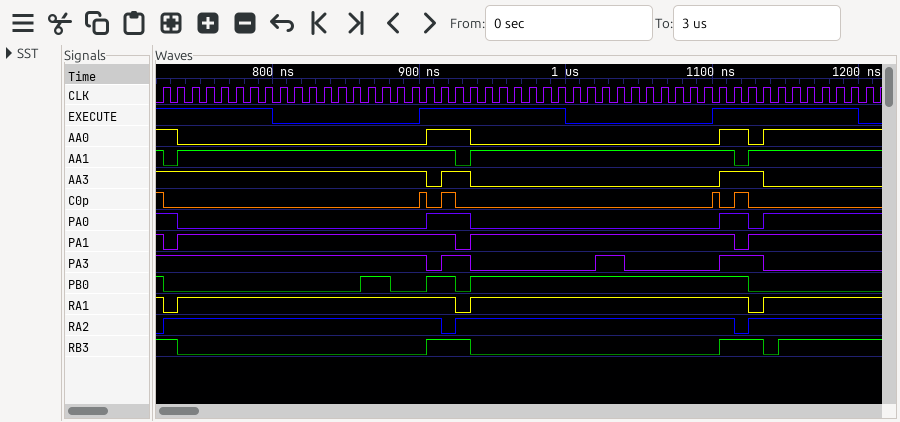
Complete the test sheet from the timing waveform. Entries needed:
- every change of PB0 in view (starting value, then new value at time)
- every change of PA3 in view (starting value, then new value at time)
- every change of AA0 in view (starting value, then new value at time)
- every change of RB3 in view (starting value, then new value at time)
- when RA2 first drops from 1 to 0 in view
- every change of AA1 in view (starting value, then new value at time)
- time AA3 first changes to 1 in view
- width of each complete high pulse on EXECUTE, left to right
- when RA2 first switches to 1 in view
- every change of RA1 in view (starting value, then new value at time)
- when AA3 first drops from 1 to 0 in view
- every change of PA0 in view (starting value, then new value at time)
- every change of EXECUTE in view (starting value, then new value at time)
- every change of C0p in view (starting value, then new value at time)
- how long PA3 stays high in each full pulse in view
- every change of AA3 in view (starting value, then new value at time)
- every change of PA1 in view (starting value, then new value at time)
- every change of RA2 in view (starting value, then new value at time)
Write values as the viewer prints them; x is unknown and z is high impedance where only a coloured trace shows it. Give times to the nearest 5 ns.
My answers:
1, 0 at 725 ns, 1 at 860 ns, 0 at 880 ns, 1 at 905 ns, 0 at 925 ns, 1 at 935 ns, 0 at 1125 ns
1, 0 at 905 ns, 1 at 915 ns, 0 at 935 ns, 1 at 1020 ns, 0 at 1040 ns, 1 at 1105 ns, 0 at 1135 ns
1, 0 at 735 ns, 1 at 905 ns, 0 at 935 ns, 1 at 1105 ns, 0 at 1125 ns, 1 at 1135 ns
1, 0 at 735 ns, 1 at 905 ns, 0 at 935 ns, 1 at 1105 ns, 0 at 1135 ns, 1 at 1145 ns
915 ns
1, 0 at 725 ns, 1 at 735 ns, 0 at 925 ns, 1 at 935 ns, 0 at 1115 ns, 1 at 1125 ns
915 ns
100 ns, 100 ns
725 ns
1, 0 at 725 ns, 1 at 735 ns, 0 at 925 ns, 1 at 935 ns, 0 at 1125 ns, 1 at 1135 ns
905 ns
1, 0 at 735 ns, 1 at 905 ns, 0 at 935 ns, 1 at 1105 ns, 0 at 1125 ns, 1 at 1135 ns
1, 0 at 800 ns, 1 at 900 ns, 0 at 1000 ns, 1 at 1100 ns, 0 at 1200 ns
1, 0 at 725 ns, 1 at 900 ns, 0 at 905 ns, 1 at 915 ns, 0 at 925 ns, 1 at 1100 ns, 0 at 1105 ns, 1 at 1115 ns, 0 at 1125 ns
20 ns, 20 ns, 30 ns
1, 0 at 905 ns, 1 at 915 ns, 0 at 935 ns, 1 at 1105 ns, 0 at 1135 ns
1, 0 at 725 ns, 1 at 735 ns, 0 at 925 ns, 1 at 935 ns, 0 at 1115 ns, 1 at 1125 ns
0, 1 at 725 ns, 0 at 915 ns, 1 at 925 ns, 0 at 1115 ns, 1 at 1125 ns
